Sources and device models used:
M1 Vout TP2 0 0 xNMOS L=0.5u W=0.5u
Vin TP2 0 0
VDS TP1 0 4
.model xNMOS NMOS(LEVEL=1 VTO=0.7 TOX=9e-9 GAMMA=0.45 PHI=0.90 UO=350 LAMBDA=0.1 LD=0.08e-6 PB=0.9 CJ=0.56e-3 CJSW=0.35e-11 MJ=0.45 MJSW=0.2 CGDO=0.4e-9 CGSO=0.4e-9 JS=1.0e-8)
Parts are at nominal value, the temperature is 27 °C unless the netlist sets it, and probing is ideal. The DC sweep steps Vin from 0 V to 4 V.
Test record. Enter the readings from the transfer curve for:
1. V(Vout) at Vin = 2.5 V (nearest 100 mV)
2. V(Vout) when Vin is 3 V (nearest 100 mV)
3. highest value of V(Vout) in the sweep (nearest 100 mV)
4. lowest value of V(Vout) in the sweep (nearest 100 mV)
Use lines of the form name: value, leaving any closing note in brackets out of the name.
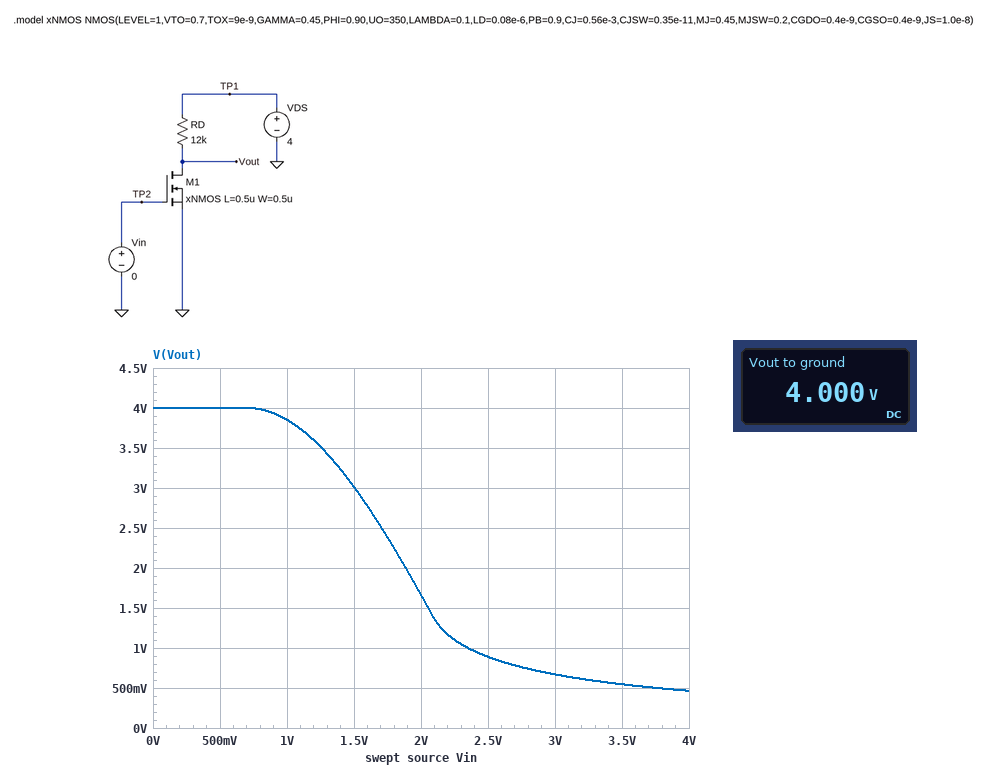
V(Vout) at Vin = 2.5 V: 900 mV
V(Vout) when Vin is 3 V: 700 mV
highest value of V(Vout) in the sweep: 4.0 V
lowest value of V(Vout) in the sweep: 500 mV
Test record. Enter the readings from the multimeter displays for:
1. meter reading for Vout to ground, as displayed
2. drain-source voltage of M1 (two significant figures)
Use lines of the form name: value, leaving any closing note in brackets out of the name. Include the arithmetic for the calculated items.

meter reading for Vout to ground, as displayed: 4.000 V
drain-source voltage of M1: 4 V = 4.0 V
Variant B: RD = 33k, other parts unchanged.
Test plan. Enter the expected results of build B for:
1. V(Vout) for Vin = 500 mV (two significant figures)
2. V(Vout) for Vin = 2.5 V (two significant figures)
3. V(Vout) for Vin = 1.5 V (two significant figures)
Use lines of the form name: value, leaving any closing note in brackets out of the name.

V(Vout) for Vin = 500 mV: 4.0 V
V(Vout) for Vin = 2.5 V: 330 mV
V(Vout) for Vin = 1.5 V: 1.6 V
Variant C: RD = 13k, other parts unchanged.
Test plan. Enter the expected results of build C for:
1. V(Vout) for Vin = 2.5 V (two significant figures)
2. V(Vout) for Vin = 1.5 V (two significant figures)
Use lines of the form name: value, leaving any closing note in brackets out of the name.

V(Vout) for Vin = 2.5 V: 820 mV
V(Vout) for Vin = 1.5 V: 2.9 V
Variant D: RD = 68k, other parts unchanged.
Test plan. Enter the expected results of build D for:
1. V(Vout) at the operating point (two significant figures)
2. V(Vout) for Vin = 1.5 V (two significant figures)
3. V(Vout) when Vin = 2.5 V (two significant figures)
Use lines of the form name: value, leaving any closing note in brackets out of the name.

V(Vout) at the operating point: 4.0 V
V(Vout) for Vin = 1.5 V: 440 mV
V(Vout) when Vin = 2.5 V: 160 mV
